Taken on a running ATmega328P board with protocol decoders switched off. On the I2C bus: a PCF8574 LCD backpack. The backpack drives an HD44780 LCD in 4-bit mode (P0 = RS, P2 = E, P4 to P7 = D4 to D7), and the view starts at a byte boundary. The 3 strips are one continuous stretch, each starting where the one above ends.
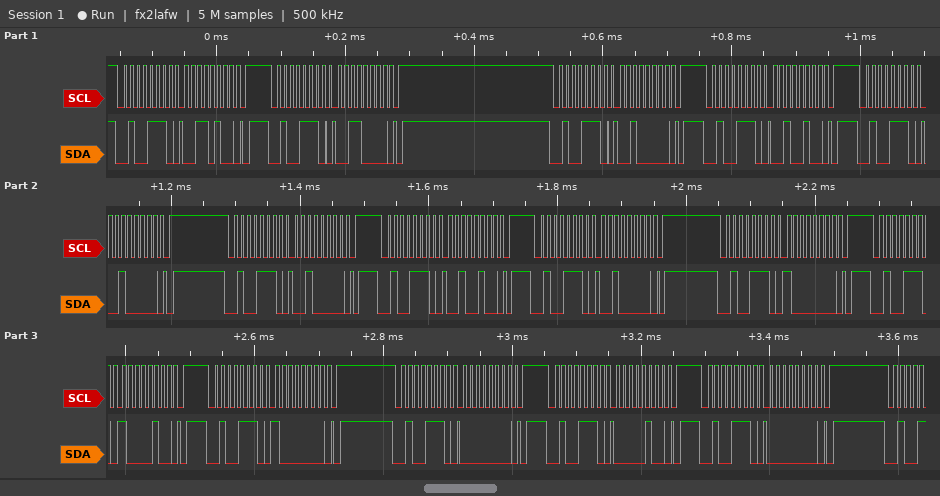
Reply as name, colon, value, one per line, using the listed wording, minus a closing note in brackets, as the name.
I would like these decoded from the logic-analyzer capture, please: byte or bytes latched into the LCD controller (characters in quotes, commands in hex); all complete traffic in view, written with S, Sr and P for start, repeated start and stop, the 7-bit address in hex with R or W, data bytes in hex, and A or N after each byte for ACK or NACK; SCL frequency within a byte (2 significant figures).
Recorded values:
byte or bytes latched into the LCD controller: 0x28
all complete traffic in view, written with S, Sr and P for start, repeated start and stop, the 7-bit address in hex with R or W, data bytes in hex, and A or N after each byte for ACK or NACK: S 27W A 34 A P S 27W A 30 A P S 27W A 20 A P S 27W A 24 A P S 27W A 20 A P S 27W A 20 A P S 27W A 24 A P S 27W A 20 A P S 27W A 80 A P S 27W A 84 A P S 27W A 80 A P S 27W A 00 A P S 27W A 04 A P S 27W A 00 A P
SCL frequency within a byte: 100 kHz
